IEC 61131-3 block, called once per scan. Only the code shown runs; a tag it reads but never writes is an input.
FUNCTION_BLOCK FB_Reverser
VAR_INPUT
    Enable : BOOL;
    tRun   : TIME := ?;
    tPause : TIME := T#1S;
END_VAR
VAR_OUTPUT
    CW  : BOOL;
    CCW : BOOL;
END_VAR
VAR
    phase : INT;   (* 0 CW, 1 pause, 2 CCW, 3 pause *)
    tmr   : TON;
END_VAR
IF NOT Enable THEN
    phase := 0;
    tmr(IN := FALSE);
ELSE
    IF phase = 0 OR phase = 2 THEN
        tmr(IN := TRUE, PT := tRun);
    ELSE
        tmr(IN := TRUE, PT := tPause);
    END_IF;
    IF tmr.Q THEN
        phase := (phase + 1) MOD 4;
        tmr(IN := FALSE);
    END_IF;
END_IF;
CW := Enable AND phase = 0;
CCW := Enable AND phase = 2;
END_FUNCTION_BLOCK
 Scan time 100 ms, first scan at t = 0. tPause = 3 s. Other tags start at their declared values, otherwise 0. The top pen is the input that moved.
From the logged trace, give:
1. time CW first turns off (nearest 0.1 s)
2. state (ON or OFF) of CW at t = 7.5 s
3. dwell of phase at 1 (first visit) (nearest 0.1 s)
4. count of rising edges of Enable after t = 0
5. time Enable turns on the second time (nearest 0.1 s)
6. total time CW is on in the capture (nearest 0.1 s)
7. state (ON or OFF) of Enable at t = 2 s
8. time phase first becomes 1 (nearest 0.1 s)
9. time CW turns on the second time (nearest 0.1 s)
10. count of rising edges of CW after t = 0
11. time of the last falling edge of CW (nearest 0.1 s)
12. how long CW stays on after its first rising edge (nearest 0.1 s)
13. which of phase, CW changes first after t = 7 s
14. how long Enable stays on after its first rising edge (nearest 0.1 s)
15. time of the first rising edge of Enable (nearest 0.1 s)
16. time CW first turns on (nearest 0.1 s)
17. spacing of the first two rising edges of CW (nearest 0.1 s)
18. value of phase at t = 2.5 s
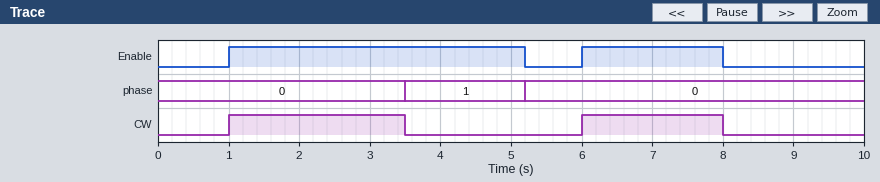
3.5 s
ON
1.7 s
2
6.0 s
4.5 s
ON
3.5 s
6.0 s
2
8.0 s
2.5 s
CW
4.2 s
1.0 s
1.0 s
5.0 s
0
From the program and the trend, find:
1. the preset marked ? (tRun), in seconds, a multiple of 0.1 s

2.5 s
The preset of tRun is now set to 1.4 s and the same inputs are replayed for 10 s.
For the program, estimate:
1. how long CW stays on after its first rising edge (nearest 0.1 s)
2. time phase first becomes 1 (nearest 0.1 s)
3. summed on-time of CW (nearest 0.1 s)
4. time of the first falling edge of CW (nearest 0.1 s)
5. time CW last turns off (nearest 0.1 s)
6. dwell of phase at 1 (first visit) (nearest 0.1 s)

1.4 s
2.4 s
2.8 s
2.4 s
7.4 s
2.8 s
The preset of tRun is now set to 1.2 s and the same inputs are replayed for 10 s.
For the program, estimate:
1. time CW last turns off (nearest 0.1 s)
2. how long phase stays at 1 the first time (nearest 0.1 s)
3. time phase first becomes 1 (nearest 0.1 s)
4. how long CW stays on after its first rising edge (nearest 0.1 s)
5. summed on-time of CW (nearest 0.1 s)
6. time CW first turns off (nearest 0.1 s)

7.2 s
3.0 s
2.2 s
1.2 s
2.4 s
2.2 s
